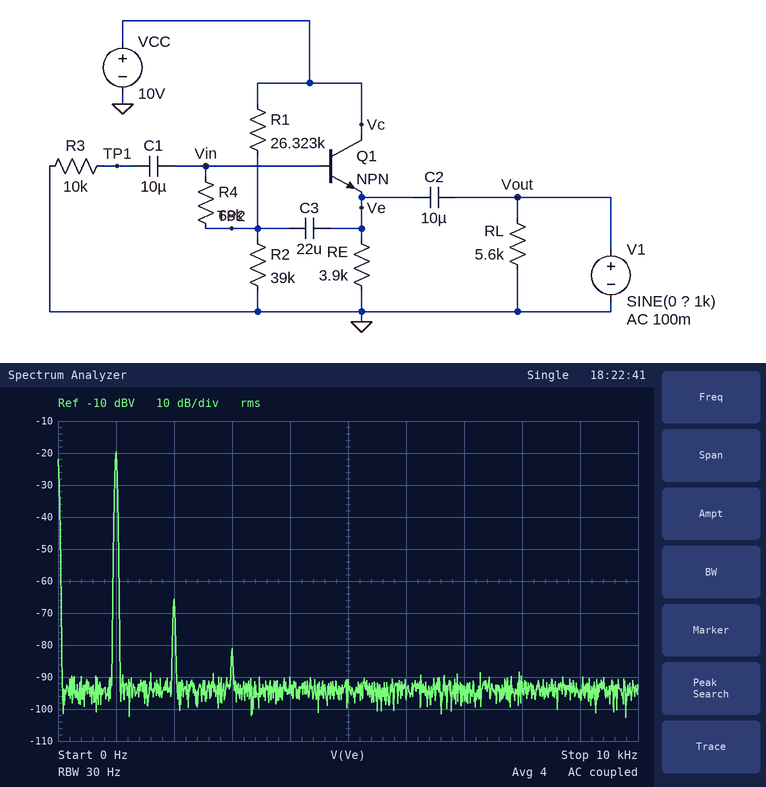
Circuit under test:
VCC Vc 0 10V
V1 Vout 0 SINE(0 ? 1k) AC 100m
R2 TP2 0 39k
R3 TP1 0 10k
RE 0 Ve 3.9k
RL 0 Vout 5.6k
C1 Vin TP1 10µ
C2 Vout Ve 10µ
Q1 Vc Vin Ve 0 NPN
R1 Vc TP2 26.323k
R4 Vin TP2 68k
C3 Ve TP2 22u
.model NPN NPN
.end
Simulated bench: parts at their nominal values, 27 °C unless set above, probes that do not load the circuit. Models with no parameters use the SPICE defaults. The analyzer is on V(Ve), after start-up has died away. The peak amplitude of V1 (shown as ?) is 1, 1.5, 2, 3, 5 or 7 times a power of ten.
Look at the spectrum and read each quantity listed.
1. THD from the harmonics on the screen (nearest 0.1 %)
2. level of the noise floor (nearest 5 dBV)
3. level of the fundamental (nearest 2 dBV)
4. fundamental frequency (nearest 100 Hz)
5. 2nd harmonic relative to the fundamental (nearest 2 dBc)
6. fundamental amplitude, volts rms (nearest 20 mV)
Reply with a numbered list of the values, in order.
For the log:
1. 0.5 %
2. -95 dBV
3. -20 dBV
4. 1.0 kHz
5. -46 dBc
6. 100 mV
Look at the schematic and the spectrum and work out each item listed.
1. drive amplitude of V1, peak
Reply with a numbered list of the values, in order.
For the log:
1. 150 mV
